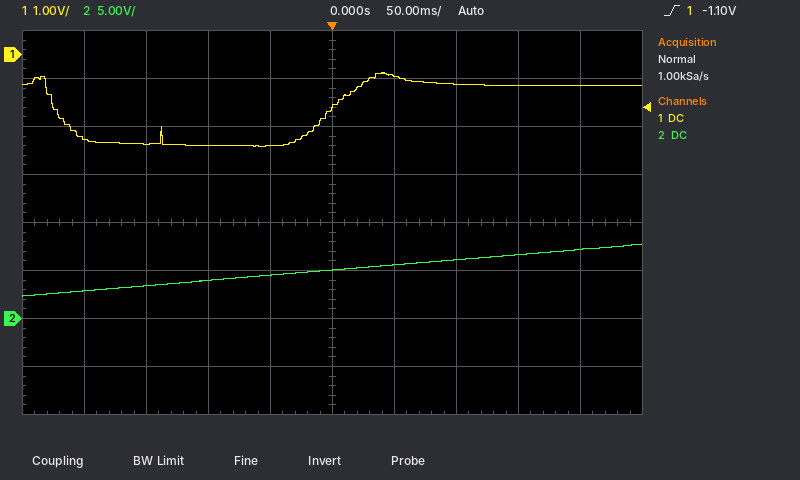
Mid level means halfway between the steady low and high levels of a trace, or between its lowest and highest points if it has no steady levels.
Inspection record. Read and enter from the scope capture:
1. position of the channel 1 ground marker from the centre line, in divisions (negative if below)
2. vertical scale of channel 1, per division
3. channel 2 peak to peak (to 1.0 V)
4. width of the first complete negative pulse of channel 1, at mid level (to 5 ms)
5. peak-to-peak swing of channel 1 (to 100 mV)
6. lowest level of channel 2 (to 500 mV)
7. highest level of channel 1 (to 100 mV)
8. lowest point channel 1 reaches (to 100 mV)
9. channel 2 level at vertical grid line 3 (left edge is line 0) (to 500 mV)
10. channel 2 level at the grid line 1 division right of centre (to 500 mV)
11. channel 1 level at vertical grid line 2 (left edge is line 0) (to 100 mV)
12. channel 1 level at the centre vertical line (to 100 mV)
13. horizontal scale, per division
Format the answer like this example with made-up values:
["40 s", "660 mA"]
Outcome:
["+3.5 div", "1 V", "5.0 V", "215 ms", "1.5 V", "2.5 V", "-400 mV", "-1.9 V", "4.0 V", "5.5 V", "-1.9 V", "-1.1 V", "50 ms"]
